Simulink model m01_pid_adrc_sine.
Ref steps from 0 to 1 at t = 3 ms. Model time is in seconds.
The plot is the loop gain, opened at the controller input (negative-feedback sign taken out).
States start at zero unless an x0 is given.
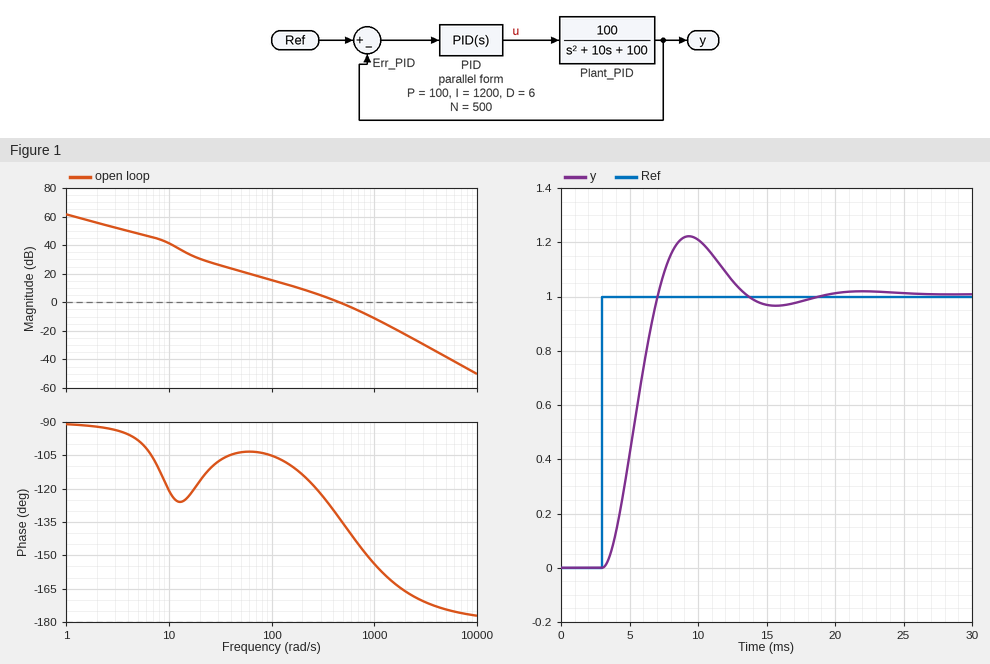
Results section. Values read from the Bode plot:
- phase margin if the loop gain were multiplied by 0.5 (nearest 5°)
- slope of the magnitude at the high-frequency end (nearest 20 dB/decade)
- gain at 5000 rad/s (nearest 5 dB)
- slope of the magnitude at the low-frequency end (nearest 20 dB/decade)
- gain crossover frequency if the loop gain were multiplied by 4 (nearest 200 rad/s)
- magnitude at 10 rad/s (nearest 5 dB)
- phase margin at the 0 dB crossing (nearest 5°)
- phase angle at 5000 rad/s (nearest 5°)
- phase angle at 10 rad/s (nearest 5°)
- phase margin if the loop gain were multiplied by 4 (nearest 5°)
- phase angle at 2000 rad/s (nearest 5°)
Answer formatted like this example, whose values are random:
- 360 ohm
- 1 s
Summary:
- 60°
- -40 dB/decade
- -40 dB
- -20 dB/decade
- 1000 rad/s
- 40 dB
- 45°
- -175°
- -120°
- 25°
- -165°
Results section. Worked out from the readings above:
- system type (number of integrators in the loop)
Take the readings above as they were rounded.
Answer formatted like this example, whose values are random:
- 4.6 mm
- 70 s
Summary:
- 1
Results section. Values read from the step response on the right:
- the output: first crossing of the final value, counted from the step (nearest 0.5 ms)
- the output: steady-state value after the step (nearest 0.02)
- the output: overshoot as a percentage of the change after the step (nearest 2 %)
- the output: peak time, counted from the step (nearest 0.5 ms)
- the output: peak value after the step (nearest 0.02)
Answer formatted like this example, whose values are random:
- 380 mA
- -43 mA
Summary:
- 4.0 ms
- 1.00
- 22 %
- 6.5 ms
- 1.22
